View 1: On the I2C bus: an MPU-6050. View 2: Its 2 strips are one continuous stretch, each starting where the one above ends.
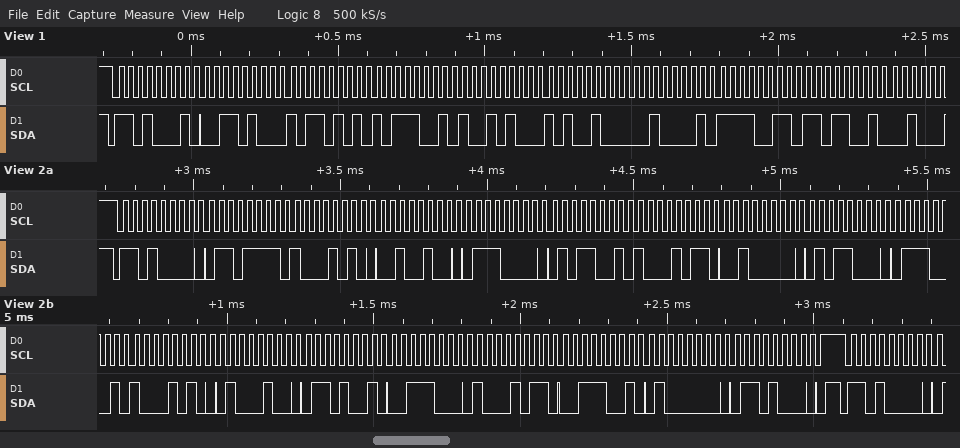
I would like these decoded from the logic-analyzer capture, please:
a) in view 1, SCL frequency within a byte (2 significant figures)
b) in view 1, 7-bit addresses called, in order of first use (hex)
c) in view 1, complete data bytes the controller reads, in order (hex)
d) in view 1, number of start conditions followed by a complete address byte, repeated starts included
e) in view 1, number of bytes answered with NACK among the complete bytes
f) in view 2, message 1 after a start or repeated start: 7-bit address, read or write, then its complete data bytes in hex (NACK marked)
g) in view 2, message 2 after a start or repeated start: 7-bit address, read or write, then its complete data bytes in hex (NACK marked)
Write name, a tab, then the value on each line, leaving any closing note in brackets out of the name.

in view 1, SCL frequency within a byte	31 kHz
in view 1, 7-bit addresses called, in order of first use	0x68
in view 1, complete data bytes the controller reads, in order	34 B5 B9 94 A4 21 F3 D9
in view 1, number of start conditions followed by a complete address byte, repeated starts included	1
in view 1, number of bytes answered with NACK among the complete bytes	0
in view 2, message 1 after a start or repeated start: 7-bit address, read or write, then its complete data bytes in hex	0x68 write: 6F 8A 24 70 59 8B 20 58 71 8A 44 69 38 8B 39 40 68
in view 2, message 2 after a start or repeated start: 7-bit address, read or write, then its complete data bytes in hex	0x68 write
